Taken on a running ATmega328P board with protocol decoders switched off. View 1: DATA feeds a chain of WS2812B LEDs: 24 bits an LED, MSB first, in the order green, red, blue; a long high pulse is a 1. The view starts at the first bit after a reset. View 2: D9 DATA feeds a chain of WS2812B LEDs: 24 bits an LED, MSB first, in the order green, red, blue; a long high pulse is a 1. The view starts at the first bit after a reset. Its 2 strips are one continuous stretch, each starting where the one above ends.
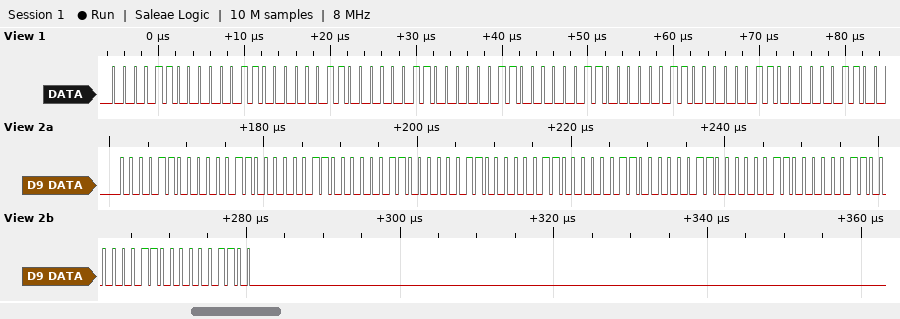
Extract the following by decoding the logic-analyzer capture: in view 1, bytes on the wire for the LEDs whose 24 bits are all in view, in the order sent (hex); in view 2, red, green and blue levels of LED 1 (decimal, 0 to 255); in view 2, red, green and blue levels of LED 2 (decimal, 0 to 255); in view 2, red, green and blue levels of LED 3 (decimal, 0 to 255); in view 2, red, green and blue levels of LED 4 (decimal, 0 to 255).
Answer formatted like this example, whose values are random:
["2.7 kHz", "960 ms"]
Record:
["0C 0C 0C 0C 0C 0C 0C 0C 0C", "12, 12, 12", "12, 12, 12", "12, 12, 12", "12, 12, 12"]
